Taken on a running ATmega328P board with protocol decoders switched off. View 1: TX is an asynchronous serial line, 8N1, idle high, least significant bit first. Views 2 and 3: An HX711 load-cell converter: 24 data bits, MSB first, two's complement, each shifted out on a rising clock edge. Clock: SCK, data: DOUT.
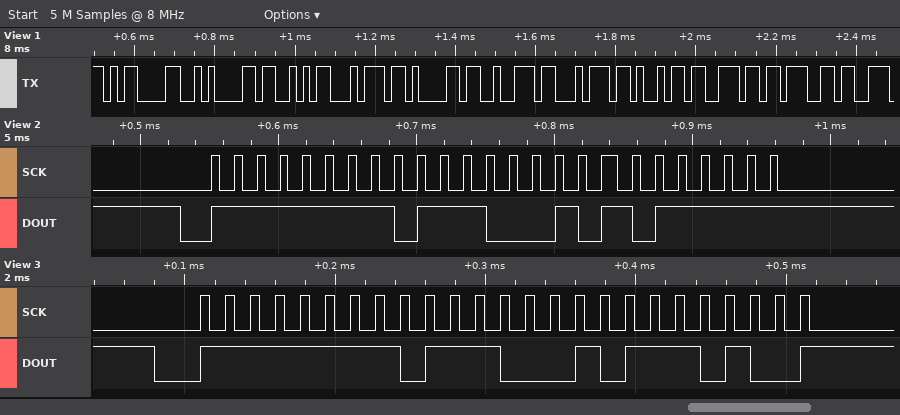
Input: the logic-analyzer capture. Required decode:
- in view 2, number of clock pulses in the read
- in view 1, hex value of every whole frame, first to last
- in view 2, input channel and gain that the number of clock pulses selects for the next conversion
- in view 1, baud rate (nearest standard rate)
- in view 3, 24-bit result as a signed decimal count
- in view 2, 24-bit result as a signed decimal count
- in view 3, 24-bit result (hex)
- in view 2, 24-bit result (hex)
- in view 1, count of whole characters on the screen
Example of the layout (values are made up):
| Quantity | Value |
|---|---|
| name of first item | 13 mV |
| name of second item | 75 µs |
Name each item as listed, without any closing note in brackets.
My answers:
| Quantity | Value |
|---|---|
| in view 2, number of clock pulses in the read | 25 |
| in view 1, hex value of every whole frame, first to last | 0D 0A 53 74 61 72 74 69 6E 67 |
| in view 2, input channel and gain that the number of clock pulses selects for the next conversion | channel A, gain 128 |
| in view 1, baud rate | 57600 baud |
| in view 3, 24-bit result as a signed decimal count | -36492 |
| in view 2, 24-bit result as a signed decimal count | -36513 |
| in view 3, 24-bit result | 0xFF7174 |
| in view 2, 24-bit result | 0xFF715F |
| in view 1, count of whole characters on the screen | 10 |
